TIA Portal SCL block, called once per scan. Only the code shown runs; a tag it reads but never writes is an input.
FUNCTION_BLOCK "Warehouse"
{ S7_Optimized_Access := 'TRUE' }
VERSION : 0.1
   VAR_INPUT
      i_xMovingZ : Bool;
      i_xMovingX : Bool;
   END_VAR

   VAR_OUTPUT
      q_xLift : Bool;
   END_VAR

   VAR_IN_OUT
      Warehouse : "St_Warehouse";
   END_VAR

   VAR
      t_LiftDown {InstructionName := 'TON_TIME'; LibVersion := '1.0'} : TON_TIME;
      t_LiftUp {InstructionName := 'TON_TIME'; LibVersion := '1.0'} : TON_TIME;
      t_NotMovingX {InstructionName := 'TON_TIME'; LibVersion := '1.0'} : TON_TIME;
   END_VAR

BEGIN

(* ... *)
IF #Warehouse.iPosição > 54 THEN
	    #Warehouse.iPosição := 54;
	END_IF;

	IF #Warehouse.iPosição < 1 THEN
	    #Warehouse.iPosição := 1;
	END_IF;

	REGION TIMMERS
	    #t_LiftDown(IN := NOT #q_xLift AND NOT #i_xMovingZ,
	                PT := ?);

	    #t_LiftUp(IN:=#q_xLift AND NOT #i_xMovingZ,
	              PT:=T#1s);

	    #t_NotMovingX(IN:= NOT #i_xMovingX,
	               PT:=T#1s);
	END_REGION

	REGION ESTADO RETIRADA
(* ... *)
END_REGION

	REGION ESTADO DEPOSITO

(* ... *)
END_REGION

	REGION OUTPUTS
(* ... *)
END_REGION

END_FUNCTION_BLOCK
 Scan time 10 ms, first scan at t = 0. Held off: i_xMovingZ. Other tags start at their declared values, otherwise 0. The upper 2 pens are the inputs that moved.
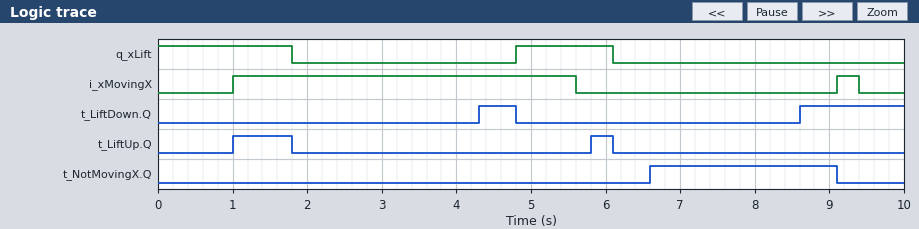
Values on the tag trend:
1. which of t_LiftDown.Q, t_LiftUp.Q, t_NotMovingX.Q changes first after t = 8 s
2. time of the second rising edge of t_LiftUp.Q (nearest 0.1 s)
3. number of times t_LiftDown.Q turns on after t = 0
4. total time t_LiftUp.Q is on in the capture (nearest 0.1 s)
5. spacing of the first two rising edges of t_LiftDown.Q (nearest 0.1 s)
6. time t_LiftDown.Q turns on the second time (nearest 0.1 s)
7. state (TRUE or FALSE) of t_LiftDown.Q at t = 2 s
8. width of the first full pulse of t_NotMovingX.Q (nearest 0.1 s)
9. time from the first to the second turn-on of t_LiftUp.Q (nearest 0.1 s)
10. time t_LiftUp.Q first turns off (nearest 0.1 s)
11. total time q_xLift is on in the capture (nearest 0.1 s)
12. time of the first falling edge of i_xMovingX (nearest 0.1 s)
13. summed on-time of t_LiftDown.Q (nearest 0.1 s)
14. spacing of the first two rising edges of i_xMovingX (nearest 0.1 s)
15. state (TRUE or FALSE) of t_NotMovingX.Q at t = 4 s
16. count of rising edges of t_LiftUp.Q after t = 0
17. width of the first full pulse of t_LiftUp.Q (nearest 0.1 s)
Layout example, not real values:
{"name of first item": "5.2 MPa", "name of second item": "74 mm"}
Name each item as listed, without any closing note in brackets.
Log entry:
{"which of t_LiftDown.Q, t_LiftUp.Q, t_NotMovingX.Q changes first after t = 8 s": "t_LiftDown.Q", "time of the second rising edge of t_LiftUp.Q": "5.8 s", "number of times t_LiftDown.Q turns on after t = 0": "2", "total time t_LiftUp.Q is on in the capture": "1.1 s", "spacing of the first two rising edges of t_LiftDown.Q": "4.3 s", "time t_LiftDown.Q turns on the second time": "8.6 s", "state (TRUE or FALSE) of t_LiftDown.Q at t = 2 s": "FALSE", "width of the first full pulse of t_NotMovingX.Q": "2.5 s", "time from the first to the second turn-on of t_LiftUp.Q": "4.8 s", "time t_LiftUp.Q first turns off": "1.8 s", "total time q_xLift is on in the capture": "3.1 s", "time of the first falling edge of i_xMovingX": "5.6 s", "summed on-time of t_LiftDown.Q": "1.9 s", "spacing of the first two rising edges of i_xMovingX": "8.1 s", "state (TRUE or FALSE) of t_NotMovingX.Q at t = 4 s": "FALSE", "count of rising edges of t_LiftUp.Q after t = 0": "2", "width of the first full pulse of t_LiftUp.Q": "0.8 s"}
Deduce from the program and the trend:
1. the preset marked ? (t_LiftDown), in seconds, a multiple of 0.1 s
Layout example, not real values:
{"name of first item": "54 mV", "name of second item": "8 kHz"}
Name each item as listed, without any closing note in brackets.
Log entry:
{"the preset marked ? (t_LiftDown), in seconds, a multiple of 0.1 s": "2.5 s"}
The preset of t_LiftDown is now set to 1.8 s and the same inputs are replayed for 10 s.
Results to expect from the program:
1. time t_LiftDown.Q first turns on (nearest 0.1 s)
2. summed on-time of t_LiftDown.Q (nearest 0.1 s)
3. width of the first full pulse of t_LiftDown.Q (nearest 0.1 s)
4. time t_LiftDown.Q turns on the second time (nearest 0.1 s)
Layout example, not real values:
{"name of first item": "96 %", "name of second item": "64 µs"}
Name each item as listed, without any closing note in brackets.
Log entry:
{"time t_LiftDown.Q first turns on": "3.6 s", "summed on-time of t_LiftDown.Q": "3.3 s", "width of the first full pulse of t_LiftDown.Q": "1.2 s", "time t_LiftDown.Q turns on the second time": "7.9 s"}
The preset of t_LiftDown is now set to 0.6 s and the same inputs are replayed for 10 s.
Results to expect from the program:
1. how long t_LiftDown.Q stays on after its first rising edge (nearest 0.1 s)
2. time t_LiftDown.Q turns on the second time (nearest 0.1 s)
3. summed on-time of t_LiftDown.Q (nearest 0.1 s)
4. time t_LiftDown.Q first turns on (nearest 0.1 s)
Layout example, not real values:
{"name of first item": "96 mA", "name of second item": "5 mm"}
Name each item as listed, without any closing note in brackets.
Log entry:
{"how long t_LiftDown.Q stays on after its first rising edge": "2.4 s", "time t_LiftDown.Q turns on the second time": "6.7 s", "summed on-time of t_LiftDown.Q": "5.7 s", "time t_LiftDown.Q first turns on": "2.4 s"}
